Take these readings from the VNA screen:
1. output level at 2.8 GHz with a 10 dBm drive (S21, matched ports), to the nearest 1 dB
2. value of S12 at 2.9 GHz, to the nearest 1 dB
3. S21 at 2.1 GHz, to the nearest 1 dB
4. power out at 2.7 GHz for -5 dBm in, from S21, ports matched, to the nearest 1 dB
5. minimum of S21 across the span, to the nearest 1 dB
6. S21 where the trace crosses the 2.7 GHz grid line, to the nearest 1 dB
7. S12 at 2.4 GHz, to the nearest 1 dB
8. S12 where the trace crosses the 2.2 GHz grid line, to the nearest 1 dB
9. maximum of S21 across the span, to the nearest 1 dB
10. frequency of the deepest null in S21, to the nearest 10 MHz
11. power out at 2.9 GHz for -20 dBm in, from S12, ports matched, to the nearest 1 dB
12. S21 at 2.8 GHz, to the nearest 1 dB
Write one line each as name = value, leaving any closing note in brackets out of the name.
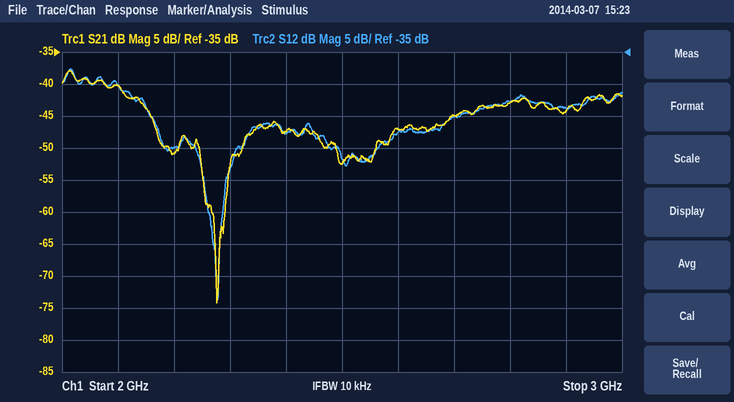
output level at 2.8 GHz with a 10 dBm drive (S21, matched ports), to the nearest 1 dB = -33 dBm
value of S12 at 2.9 GHz, to the nearest 1 dB = -44 dB
S21 at 2.1 GHz, to the nearest 1 dB = -40 dB
power out at 2.7 GHz for -5 dBm in, from S21, ports matched, to the nearest 1 dB = -50 dBm
minimum of S21 across the span, to the nearest 1 dB = -74 dB
S21 where the trace crosses the 2.7 GHz grid line, to the nearest 1 dB = -45 dB
S12 at 2.4 GHz, to the nearest 1 dB = -48 dB
S12 where the trace crosses the 2.2 GHz grid line, to the nearest 1 dB = -50 dB
maximum of S21 across the span, to the nearest 1 dB = -38 dB
frequency of the deepest null in S21, to the nearest 10 MHz = 2.28 GHz
power out at 2.9 GHz for -20 dBm in, from S12, ports matched, to the nearest 1 dB = -64 dBm
S21 at 2.8 GHz, to the nearest 1 dB = -43 dB
